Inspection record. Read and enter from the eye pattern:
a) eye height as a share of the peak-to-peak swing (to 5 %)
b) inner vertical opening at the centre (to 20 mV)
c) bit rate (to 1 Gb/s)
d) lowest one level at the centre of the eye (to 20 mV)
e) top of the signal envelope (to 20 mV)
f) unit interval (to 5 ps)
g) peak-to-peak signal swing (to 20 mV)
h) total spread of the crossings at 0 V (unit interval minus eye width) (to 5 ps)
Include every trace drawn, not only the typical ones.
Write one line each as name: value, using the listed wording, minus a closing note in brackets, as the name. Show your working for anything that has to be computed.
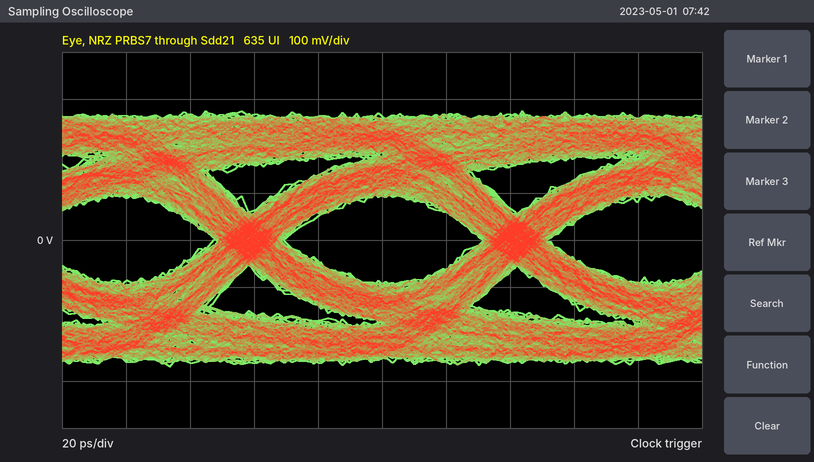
eye height as a share of the peak-to-peak swing: 180 mV / 540 mV ≈ 33.3 %, so 35 % to the nearest 5 %
inner vertical opening at the centre: 180 mV
bit rate: 12 Gb/s
lowest one level at the centre of the eye: 100 mV
top of the signal envelope: 280 mV
unit interval: 85 ps
peak-to-peak signal swing: 540 mV
total spread of the crossings at 0 V (unit interval minus eye width): 20 ps
